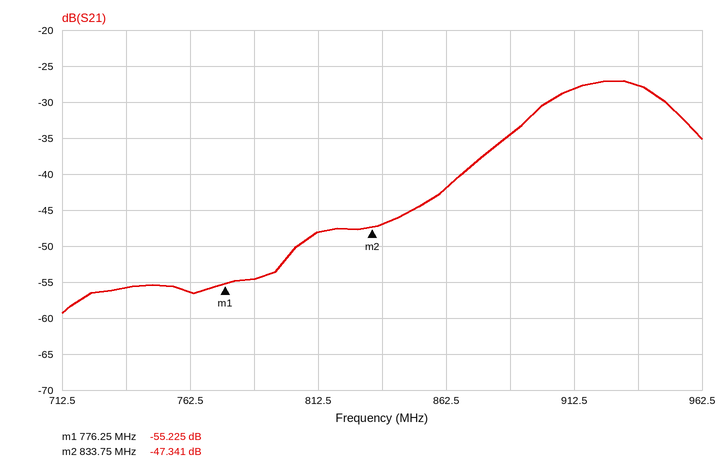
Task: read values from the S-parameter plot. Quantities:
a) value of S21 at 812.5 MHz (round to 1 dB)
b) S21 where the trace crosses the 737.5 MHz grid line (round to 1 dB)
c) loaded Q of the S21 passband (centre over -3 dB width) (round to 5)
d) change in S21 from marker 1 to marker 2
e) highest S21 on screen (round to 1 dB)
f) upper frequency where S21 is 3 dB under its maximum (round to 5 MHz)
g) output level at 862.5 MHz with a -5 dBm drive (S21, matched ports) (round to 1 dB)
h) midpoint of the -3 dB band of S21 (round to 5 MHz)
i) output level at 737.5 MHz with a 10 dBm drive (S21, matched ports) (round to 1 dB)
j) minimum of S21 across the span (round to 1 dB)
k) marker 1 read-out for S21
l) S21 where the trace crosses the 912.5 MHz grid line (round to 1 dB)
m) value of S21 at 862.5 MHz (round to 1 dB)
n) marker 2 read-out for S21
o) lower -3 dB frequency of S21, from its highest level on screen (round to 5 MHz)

-48 dB
-56 dB
20
7.884 dB
-27 dB
950 MHz
-47 dBm
925 MHz
-46 dBm
-59 dB
-55.225 dB
-28 dB
-42 dB
-47.341 dB
900 MHz
